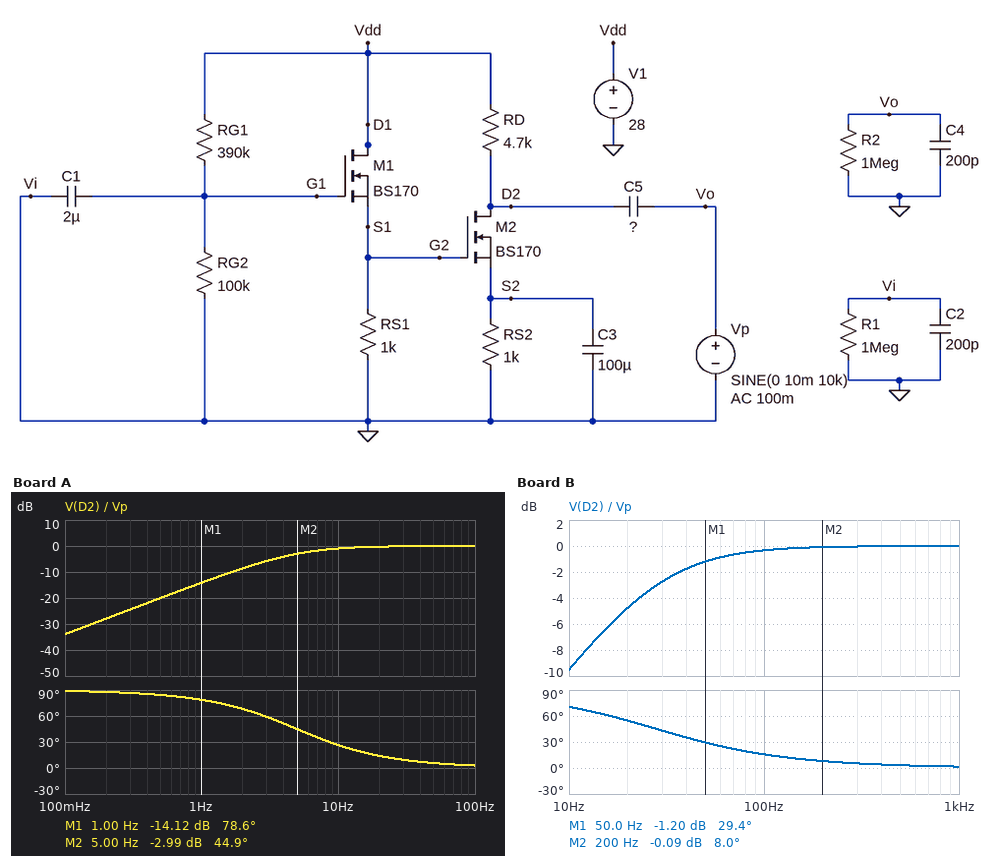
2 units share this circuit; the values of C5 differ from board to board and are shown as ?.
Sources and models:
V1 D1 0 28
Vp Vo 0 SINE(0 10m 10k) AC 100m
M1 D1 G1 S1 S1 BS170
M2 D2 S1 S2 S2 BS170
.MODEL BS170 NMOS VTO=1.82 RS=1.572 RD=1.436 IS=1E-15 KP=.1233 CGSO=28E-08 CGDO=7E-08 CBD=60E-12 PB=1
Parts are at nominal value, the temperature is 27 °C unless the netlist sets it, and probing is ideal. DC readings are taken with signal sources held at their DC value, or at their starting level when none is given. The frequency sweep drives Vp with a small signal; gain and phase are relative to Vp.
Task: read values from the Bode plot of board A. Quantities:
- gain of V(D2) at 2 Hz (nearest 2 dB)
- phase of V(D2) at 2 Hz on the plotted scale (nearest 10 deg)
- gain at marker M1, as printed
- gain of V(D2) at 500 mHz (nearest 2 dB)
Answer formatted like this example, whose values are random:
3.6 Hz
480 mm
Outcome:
-8 dB
70 deg
-14.12 dB
-20 dB
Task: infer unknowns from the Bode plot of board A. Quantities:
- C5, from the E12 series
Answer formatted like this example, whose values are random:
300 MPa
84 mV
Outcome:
6.8 µF
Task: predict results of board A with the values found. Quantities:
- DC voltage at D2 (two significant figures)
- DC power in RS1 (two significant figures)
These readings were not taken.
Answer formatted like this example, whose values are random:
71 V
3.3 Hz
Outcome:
20 V
13 mW
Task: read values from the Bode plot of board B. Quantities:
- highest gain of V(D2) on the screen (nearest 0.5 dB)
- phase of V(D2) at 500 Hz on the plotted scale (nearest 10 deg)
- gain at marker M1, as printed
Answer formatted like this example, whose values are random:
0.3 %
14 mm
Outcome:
0 dB
0 deg
-1.20 dB
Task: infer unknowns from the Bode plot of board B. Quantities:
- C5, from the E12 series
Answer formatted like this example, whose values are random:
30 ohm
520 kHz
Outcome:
1.2 µF
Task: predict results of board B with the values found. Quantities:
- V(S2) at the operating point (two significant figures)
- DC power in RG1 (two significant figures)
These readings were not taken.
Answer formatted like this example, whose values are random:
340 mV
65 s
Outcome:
1.7 V
1.3 mW
